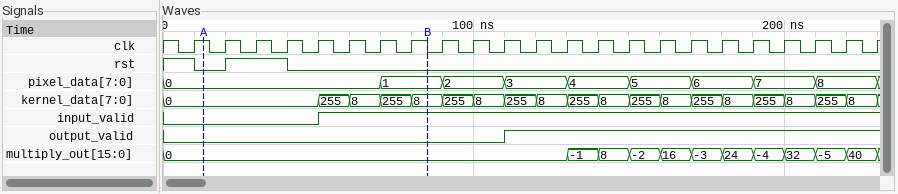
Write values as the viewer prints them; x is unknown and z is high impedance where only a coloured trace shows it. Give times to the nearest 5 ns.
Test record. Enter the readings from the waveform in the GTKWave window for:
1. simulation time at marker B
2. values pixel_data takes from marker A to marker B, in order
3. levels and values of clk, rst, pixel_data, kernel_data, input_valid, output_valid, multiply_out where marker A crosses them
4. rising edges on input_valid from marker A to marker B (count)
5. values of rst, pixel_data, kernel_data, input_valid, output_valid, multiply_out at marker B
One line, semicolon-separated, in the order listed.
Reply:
85 ns; 0, 1; clk=1, rst=0, pixel_data=0, kernel_data=0, input_valid=0, output_valid=0, multiply_out=0; 1; rst=0, pixel_data=1, kernel_data=8, input_valid=1, output_valid=0, multiply_out=0
